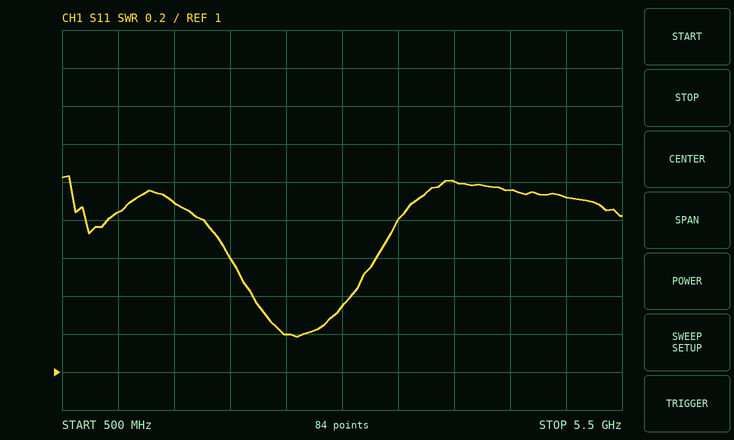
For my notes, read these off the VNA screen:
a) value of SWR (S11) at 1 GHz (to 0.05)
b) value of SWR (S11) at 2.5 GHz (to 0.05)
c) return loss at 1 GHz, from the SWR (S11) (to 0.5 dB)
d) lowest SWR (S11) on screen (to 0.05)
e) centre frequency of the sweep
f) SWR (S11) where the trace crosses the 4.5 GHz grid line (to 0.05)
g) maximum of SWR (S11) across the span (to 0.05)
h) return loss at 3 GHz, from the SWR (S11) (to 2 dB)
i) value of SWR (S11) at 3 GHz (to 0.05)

1.85
1.20
10.5 dB
1.20
3 GHz
1.95
2.05
16 dB
1.35
